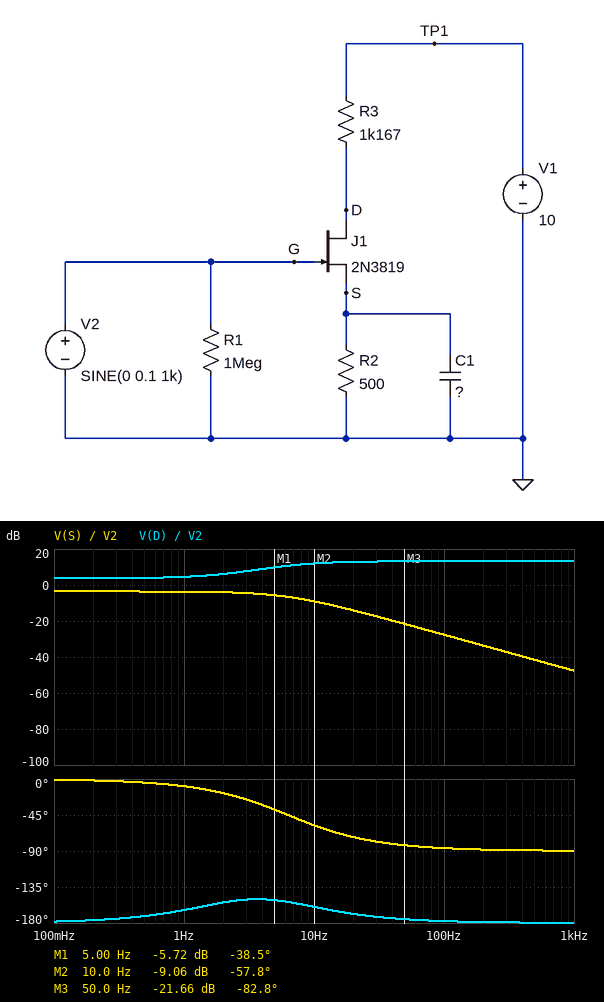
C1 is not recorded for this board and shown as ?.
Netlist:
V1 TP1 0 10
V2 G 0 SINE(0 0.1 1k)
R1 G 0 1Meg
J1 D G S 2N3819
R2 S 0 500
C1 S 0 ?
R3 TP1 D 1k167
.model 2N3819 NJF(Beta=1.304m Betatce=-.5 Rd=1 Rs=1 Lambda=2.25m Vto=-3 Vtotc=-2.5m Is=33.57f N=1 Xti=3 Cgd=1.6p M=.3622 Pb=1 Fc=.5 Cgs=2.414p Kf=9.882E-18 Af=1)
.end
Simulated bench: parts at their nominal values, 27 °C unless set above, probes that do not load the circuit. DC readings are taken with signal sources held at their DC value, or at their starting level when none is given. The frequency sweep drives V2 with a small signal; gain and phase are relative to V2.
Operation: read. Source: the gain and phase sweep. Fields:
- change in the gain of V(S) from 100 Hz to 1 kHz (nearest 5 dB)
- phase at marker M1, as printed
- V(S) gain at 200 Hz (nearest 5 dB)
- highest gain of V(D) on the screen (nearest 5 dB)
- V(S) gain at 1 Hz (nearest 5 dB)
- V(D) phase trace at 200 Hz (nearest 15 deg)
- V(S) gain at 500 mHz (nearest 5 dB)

-20 dB
-38.5 deg
-35 dB
15 dB
-5 dB
-180 deg
-5 dB
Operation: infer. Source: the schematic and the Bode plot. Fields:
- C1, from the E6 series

150 µF
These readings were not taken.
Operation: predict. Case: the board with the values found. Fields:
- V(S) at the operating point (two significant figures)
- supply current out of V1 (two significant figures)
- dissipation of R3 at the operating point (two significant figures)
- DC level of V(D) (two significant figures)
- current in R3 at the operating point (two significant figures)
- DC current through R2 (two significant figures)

1.5 V
3.0 mA
10 mW
6.5 V
3.0 mA
3.0 mA
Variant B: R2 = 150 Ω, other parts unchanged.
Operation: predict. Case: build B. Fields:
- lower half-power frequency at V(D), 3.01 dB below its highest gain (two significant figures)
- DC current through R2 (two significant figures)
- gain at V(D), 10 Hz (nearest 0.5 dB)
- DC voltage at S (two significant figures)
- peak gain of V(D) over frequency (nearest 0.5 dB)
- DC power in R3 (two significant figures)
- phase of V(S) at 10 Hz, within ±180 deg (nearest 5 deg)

8.1 Hz
5.9 mA
13.5 dB
880 mV
16.0 dB
40 mW
-40 deg
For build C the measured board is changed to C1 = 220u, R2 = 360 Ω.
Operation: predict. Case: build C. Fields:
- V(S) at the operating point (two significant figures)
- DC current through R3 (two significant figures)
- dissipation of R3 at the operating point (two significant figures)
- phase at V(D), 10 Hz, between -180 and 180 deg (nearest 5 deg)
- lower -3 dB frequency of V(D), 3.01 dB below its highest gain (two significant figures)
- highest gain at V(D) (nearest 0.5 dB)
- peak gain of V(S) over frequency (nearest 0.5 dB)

1.3 V
3.7 mA
16 mW
-165 deg
4.3 Hz
14.0 dB
-4.5 dB
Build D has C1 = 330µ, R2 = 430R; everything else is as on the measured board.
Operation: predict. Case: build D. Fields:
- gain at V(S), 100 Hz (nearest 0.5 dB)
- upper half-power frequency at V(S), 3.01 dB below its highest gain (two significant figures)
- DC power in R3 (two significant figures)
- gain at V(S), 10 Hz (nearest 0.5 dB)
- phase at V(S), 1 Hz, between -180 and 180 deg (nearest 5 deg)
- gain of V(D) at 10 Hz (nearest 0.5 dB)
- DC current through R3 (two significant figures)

-34.0 dB
3.1 Hz
13 mW
-14.5 dB
-20 deg
13.5 dB
3.3 mA
